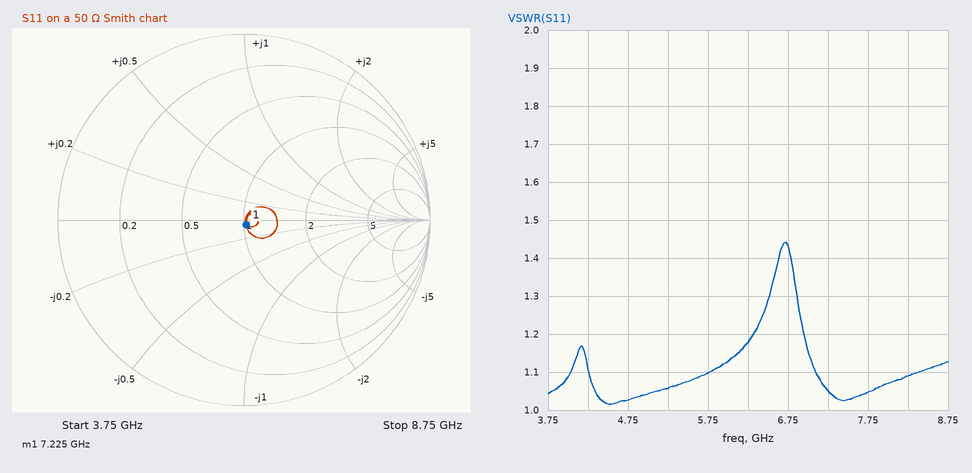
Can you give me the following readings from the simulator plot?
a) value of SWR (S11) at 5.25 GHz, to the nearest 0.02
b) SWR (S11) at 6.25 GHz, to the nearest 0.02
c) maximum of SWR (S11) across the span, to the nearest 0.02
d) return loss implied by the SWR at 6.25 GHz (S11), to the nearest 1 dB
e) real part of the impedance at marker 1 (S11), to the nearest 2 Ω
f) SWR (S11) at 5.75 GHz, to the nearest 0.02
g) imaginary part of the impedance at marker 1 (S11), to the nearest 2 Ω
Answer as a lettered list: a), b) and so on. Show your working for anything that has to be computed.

a) 1.06
b) 1.18
c) 1.44
d) −20 log10((1.18 − 1)/(1.18 + 1)) ≈ 22 dB
e) 52 Ω
f) 1.10
g) -2 Ω
